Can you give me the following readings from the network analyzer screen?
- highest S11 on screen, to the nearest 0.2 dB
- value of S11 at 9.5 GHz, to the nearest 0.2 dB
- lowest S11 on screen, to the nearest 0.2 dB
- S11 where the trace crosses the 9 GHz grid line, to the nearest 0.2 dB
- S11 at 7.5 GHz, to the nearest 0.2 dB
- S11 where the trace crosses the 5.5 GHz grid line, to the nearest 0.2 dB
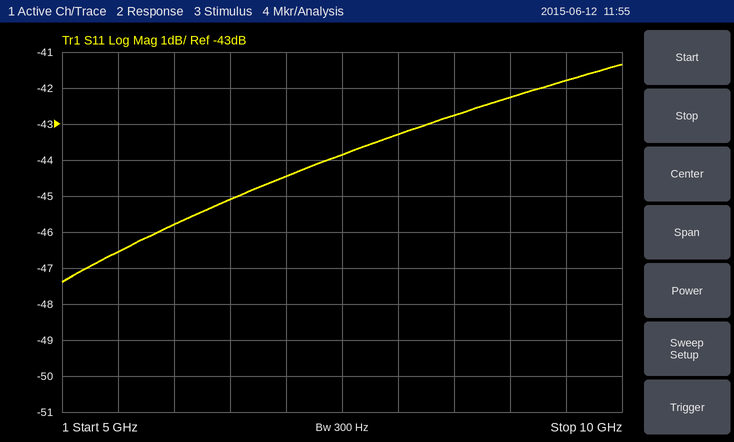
-41.4 dB
-41.8 dB
-47.4 dB
-42.2 dB
-43.8 dB
-46.6 dB
